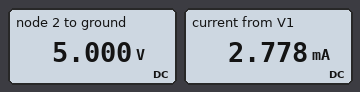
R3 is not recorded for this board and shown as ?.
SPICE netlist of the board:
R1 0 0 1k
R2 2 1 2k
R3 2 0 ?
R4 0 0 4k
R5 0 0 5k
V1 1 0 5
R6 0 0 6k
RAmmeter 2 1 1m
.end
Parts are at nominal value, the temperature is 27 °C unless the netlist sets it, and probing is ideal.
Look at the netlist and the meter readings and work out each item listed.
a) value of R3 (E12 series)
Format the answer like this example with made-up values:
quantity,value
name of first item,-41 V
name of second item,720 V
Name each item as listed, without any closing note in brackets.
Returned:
quantity,value
value of R3,1.8 kΩ
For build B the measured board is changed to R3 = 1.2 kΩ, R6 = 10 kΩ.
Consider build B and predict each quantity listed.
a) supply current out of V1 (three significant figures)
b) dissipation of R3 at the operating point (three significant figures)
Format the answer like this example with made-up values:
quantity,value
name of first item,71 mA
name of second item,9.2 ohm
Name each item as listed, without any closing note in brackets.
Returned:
quantity,value
supply current out of V1,4.17 mA
dissipation of R3 at the operating point,20.8 mW
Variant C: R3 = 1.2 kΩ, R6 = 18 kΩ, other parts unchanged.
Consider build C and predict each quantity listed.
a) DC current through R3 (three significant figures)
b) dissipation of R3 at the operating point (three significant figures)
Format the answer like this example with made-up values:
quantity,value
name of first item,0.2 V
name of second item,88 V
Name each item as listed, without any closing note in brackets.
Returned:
quantity,value
DC current through R3,4.17 mA
dissipation of R3 at the operating point,20.8 mW
